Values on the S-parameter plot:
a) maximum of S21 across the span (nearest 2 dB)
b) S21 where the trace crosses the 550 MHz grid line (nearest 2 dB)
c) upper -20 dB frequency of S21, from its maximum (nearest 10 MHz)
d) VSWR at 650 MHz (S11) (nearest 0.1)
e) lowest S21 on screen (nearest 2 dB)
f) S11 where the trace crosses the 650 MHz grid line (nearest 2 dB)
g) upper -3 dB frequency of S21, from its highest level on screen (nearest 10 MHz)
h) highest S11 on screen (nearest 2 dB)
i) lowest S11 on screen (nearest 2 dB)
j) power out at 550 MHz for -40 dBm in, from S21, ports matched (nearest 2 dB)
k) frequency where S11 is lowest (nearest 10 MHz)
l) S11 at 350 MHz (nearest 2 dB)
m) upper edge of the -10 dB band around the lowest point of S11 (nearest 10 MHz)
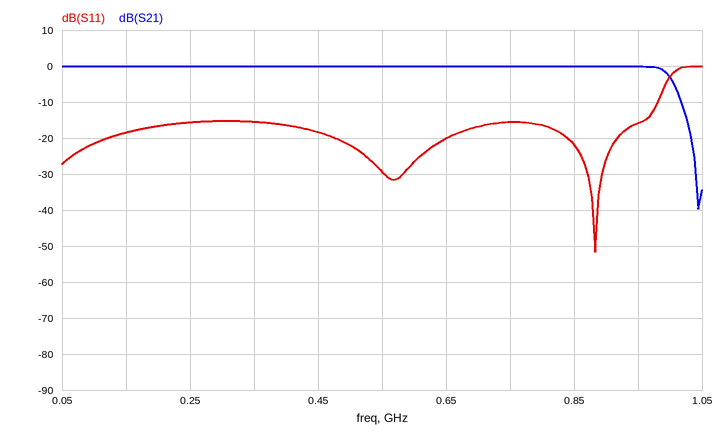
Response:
0 dB
0 dB
1.03 GHz
1.2
-40 dB
-20 dB
1.00 GHz
0 dB
-52 dB
-40 dBm
880 MHz
-16 dB
980 MHz
